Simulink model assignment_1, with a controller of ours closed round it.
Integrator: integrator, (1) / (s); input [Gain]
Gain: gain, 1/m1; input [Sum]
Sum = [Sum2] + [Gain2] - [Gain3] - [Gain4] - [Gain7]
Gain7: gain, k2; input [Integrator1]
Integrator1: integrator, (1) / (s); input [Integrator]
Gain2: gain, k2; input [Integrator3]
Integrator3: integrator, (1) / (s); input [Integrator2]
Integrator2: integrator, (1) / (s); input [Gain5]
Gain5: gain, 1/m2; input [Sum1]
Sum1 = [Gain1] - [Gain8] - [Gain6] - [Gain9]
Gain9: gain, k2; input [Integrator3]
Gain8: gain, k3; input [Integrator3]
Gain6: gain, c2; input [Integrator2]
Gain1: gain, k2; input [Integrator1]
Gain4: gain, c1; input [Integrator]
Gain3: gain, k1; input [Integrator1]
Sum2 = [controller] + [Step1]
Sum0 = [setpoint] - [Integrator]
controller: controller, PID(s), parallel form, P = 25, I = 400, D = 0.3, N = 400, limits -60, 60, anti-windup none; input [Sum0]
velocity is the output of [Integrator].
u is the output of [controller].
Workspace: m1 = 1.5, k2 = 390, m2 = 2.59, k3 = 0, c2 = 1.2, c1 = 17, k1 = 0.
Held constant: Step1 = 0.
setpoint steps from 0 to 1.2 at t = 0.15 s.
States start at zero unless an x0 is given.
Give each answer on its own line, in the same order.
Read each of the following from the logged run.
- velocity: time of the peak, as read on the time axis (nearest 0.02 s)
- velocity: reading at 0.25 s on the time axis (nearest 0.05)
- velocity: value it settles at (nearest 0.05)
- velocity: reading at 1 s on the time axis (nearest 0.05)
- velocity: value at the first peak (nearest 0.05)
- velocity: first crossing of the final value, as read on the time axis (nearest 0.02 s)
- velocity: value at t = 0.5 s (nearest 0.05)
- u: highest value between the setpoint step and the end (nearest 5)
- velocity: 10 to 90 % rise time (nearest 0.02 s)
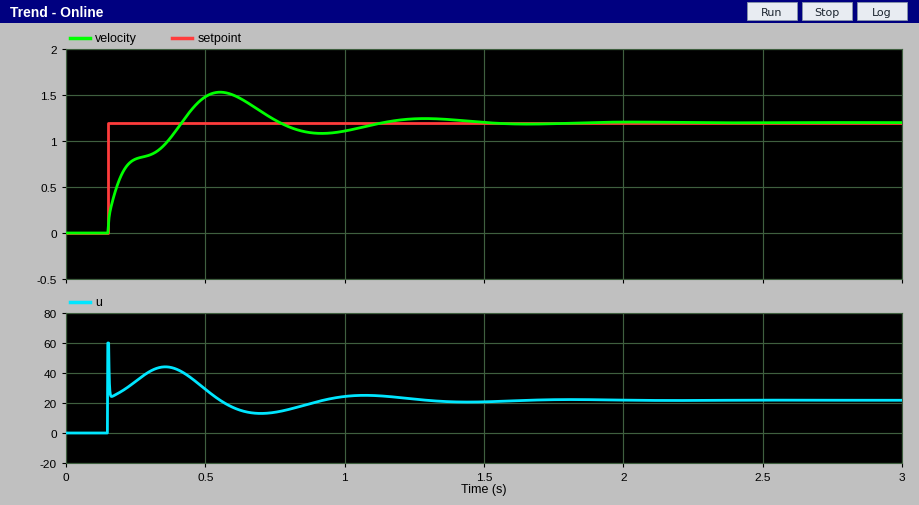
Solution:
0.56 s
0.80
1.20
1.10
1.55
0.42 s
1.50
60
0.24 s
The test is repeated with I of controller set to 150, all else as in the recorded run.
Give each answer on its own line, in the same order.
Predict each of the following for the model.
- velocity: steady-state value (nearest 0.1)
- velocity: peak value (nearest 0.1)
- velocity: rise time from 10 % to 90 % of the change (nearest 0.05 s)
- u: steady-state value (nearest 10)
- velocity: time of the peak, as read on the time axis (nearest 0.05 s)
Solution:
1.2
1.3
0.30 s
20
0.60 s
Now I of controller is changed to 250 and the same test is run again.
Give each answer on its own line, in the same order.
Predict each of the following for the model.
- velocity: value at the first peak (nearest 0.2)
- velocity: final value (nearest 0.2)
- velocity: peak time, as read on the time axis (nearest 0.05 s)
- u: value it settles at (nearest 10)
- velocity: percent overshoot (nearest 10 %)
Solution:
1.4
1.2
0.60 s
20
20 %
